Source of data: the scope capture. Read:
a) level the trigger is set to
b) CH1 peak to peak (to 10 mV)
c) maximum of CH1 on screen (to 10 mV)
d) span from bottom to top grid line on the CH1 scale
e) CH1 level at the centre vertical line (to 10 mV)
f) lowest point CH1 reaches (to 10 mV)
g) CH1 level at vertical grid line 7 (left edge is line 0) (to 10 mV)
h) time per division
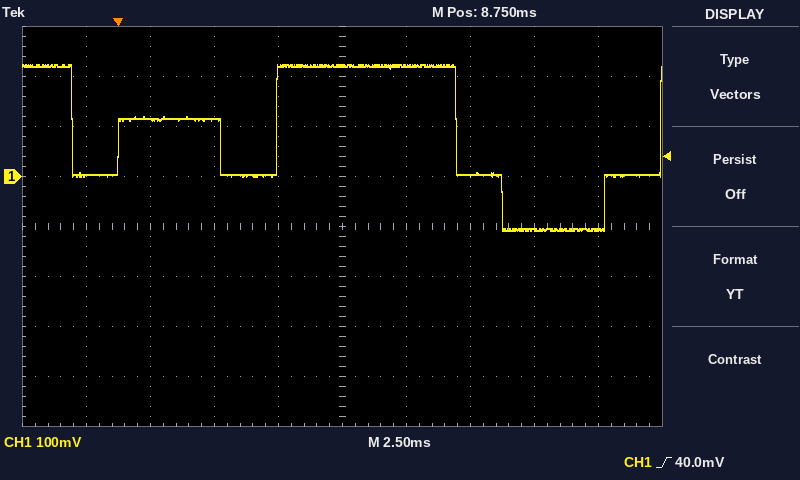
40.0 mV
330 mV
220 mV
800 mV
220 mV
-110 mV
0 mV
2.5 ms
